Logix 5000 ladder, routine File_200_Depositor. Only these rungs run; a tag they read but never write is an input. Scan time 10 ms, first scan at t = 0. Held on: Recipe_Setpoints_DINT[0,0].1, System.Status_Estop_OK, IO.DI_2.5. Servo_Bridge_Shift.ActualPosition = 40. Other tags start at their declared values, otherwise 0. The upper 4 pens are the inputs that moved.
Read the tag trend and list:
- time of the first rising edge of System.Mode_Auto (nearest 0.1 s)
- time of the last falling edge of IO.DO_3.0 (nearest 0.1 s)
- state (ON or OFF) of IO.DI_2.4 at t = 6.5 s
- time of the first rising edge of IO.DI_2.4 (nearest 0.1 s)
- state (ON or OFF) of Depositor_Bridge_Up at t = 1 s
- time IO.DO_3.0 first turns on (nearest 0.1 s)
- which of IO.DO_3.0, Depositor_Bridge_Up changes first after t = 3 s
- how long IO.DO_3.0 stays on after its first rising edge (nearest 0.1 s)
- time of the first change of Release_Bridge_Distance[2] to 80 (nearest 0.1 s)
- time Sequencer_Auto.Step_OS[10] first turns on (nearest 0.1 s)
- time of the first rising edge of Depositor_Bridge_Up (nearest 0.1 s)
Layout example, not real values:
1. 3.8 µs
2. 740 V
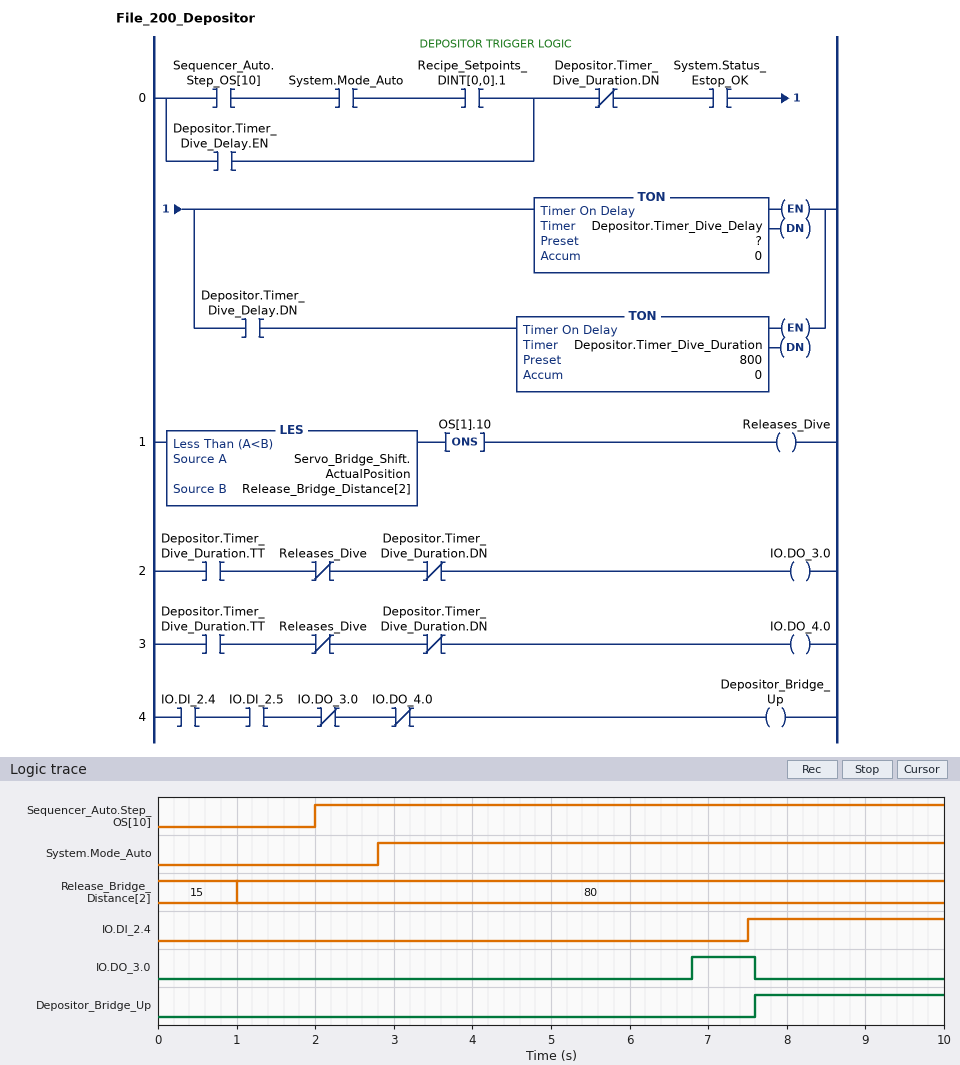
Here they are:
1. 2.8 s
2. 7.6 s
3. OFF
4. 7.5 s
5. OFF
6. 6.8 s
7. IO.DO_3.0
8. 0.8 s
9. 1.0 s
10. 2.0 s
11. 7.6 s
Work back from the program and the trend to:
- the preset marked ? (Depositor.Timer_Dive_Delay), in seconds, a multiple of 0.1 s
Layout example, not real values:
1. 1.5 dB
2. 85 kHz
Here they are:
1. 4.0 s
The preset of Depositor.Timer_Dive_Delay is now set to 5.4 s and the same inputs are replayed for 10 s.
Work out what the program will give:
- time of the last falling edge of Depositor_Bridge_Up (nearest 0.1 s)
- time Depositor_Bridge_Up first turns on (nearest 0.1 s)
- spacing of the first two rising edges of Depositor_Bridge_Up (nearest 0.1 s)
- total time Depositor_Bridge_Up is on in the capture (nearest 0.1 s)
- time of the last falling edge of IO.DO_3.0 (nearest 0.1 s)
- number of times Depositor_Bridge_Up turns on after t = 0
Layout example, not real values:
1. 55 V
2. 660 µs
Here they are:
1. 8.2 s
2. 7.5 s
3. 1.5 s
4. 1.7 s
5. 9.0 s
6. 2
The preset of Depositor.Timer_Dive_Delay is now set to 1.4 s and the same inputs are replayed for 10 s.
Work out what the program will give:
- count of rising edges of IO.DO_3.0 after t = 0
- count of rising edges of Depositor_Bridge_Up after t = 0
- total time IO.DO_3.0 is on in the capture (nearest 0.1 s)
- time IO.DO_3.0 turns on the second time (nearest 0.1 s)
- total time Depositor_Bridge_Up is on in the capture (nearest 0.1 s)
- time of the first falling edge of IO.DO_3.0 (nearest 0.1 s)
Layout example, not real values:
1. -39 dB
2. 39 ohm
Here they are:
1. 3
2. 2
3. 2.4 s
4. 6.4 s
5. 1.7 s
6. 5.0 s
